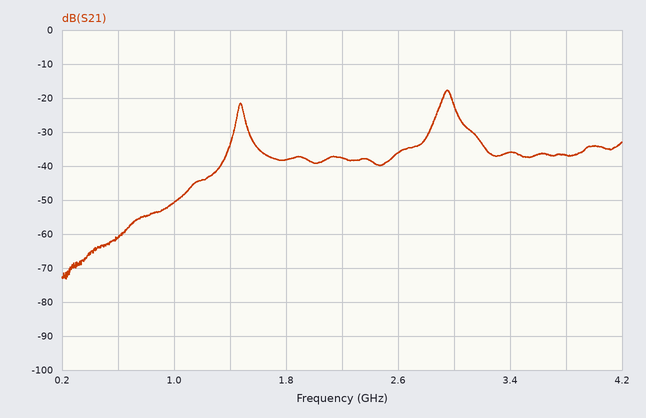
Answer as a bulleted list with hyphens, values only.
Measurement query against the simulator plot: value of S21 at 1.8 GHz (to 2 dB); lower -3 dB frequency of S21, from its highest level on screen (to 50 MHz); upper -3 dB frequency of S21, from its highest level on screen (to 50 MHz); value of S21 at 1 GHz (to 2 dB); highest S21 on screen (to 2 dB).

- -38 dB
- 2.90 GHz
- 3.00 GHz
- -50 dB
- -18 dB
